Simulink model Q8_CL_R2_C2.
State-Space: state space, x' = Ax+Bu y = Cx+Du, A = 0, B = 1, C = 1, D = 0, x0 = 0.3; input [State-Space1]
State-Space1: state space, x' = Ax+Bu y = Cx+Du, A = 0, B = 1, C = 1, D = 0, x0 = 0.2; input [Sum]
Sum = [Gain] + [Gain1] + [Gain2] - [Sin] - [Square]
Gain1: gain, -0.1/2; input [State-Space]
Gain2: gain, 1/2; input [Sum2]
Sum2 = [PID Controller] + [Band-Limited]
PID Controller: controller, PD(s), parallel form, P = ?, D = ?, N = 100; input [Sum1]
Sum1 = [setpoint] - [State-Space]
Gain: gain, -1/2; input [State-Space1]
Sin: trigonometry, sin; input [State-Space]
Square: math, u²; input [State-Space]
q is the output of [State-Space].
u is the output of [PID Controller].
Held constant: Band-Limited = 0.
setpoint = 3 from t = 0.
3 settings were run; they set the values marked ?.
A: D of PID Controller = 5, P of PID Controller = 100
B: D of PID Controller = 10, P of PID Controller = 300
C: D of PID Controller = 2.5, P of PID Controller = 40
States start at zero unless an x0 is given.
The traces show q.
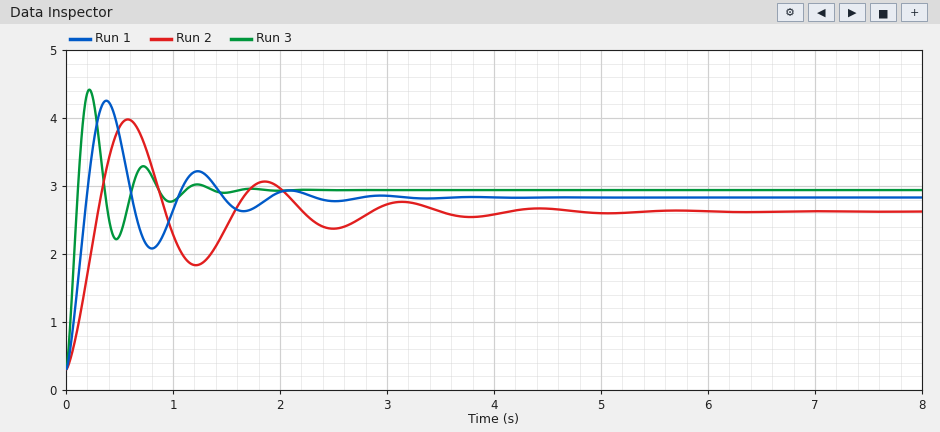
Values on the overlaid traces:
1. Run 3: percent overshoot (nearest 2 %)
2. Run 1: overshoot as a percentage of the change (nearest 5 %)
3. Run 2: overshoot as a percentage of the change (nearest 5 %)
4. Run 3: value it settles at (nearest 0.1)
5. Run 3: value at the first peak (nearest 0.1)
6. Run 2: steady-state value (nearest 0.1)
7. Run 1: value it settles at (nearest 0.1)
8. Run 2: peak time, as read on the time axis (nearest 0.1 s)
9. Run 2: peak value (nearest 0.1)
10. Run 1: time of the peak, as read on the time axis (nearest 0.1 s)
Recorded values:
56 %
55 %
60 %
2.9
4.4
2.6
2.8
0.6 s
4.0
0.4 s
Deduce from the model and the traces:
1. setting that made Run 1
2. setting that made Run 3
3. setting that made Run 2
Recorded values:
A
B
C
